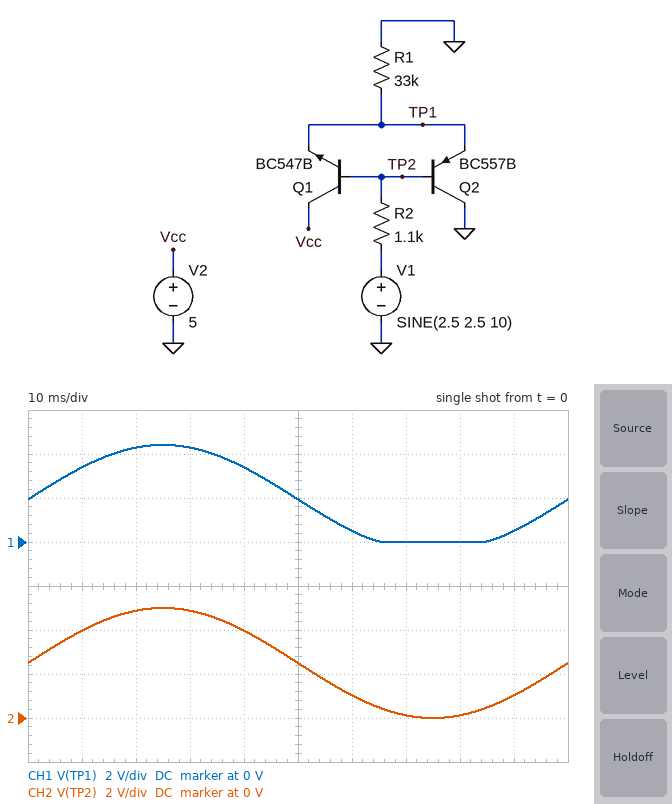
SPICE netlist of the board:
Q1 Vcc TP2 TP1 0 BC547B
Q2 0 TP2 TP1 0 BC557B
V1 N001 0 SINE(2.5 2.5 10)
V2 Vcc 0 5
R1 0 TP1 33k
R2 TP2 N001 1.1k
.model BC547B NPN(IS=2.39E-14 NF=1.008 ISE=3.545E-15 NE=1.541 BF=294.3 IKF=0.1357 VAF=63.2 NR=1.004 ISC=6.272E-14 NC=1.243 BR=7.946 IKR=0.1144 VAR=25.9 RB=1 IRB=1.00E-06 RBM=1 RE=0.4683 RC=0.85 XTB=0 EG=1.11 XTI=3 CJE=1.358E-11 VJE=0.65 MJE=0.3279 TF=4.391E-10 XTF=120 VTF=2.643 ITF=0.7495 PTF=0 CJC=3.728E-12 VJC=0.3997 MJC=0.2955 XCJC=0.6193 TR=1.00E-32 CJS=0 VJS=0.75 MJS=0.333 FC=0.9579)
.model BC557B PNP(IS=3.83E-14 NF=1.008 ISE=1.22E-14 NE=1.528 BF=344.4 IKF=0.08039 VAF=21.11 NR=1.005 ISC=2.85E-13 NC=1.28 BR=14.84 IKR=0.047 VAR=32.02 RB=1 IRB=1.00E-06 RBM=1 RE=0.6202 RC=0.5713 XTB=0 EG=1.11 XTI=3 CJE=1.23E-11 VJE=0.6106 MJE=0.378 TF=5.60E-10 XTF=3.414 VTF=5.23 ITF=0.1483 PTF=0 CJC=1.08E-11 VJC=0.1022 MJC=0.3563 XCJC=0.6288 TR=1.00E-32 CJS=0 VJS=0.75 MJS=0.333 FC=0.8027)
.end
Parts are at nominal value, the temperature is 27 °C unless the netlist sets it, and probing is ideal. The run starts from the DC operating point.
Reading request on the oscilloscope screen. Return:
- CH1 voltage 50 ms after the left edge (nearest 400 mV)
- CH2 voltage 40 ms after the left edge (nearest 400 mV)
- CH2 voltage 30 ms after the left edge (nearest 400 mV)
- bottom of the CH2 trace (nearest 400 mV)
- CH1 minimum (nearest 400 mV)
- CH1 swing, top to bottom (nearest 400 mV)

2.0 V
4.0 V
4.8 V
0 V
0 V
4.4 V
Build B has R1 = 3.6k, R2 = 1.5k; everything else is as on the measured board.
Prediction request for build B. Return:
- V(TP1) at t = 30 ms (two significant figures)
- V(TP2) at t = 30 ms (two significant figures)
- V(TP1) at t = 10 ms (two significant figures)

4.2 V
4.9 V
3.3 V
